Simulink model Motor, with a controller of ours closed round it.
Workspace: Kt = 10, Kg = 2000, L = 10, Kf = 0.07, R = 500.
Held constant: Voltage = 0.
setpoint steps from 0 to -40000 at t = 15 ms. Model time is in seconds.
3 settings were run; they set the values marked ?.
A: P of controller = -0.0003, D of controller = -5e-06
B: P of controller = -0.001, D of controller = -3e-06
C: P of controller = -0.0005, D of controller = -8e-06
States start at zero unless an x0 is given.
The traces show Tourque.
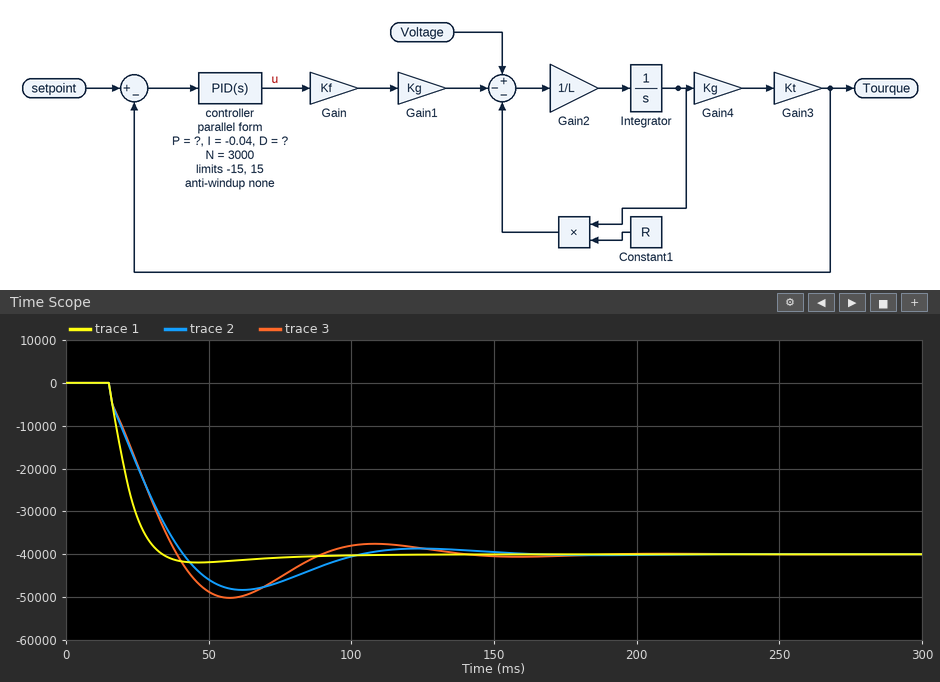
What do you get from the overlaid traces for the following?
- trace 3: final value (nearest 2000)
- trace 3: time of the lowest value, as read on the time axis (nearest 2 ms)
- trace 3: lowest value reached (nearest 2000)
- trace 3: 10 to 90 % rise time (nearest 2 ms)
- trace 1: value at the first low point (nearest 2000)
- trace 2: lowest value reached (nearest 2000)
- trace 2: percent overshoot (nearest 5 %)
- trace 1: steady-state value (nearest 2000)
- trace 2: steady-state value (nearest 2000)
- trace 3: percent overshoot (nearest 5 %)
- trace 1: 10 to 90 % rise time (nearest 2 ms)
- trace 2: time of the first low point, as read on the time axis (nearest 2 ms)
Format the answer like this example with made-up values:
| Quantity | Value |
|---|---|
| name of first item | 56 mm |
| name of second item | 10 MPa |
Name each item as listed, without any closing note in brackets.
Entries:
| Quantity | Value |
|---|---|
| trace 3: final value | -40000 |
| trace 3: time of the lowest value, as read on the time axis | 58 ms |
| trace 3: lowest value reached | -50000 |
| trace 3: 10 to 90 % rise time | 20 ms |
| trace 1: value at the first low point | -42000 |
| trace 2: lowest value reached | -48000 |
| trace 2: percent overshoot | 20 % |
| trace 1: steady-state value | -40000 |
| trace 2: steady-state value | -40000 |
| trace 3: percent overshoot | 25 % |
| trace 1: 10 to 90 % rise time | 12 ms |
| trace 2: time of the first low point, as read on the time axis | 62 ms |
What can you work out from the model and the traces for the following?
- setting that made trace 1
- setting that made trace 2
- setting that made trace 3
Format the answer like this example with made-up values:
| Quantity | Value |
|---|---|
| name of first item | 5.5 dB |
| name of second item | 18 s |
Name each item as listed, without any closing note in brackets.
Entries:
| Quantity | Value |
|---|---|
| setting that made trace 1 | B |
| setting that made trace 2 | C |
| setting that made trace 3 | A |
